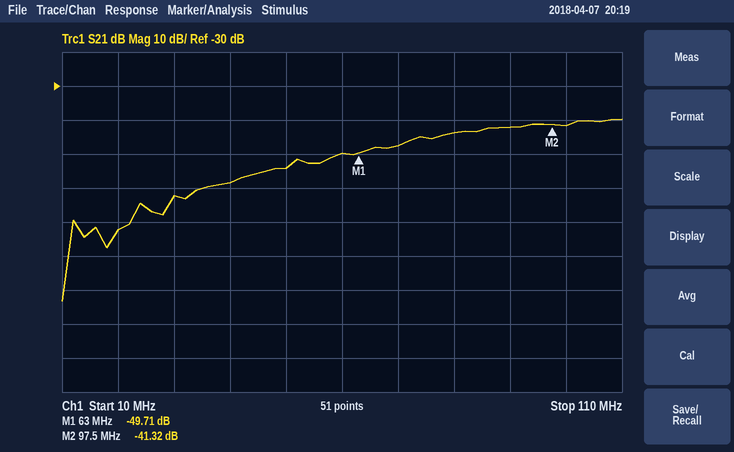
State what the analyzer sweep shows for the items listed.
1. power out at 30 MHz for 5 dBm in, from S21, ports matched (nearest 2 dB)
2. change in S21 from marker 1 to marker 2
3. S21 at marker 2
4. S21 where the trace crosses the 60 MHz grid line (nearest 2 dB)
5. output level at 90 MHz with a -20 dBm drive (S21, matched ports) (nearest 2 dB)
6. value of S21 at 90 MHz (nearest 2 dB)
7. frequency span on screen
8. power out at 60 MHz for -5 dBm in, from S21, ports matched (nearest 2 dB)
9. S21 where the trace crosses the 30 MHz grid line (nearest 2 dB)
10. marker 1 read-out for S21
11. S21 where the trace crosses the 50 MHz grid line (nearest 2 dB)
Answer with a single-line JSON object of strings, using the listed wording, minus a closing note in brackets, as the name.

{"power out at 30 MHz for 5 dBm in, from S21, ports matched": "-58 dBm", "change in S21 from marker 1 to marker 2": "8.39 dB", "S21 at marker 2": "-41.32 dB", "S21 where the trace crosses the 60 MHz grid line": "-50 dB", "output level at 90 MHz with a -20 dBm drive (S21, matched ports)": "-62 dBm", "value of S21 at 90 MHz": "-42 dB", "frequency span on screen": "100 MHz", "power out at 60 MHz for -5 dBm in, from S21, ports matched": "-54 dBm", "S21 where the trace crosses the 30 MHz grid line": "-62 dB", "marker 1 read-out for S21": "-49.71 dB", "S21 where the trace crosses the 50 MHz grid line": "-54 dB"}
